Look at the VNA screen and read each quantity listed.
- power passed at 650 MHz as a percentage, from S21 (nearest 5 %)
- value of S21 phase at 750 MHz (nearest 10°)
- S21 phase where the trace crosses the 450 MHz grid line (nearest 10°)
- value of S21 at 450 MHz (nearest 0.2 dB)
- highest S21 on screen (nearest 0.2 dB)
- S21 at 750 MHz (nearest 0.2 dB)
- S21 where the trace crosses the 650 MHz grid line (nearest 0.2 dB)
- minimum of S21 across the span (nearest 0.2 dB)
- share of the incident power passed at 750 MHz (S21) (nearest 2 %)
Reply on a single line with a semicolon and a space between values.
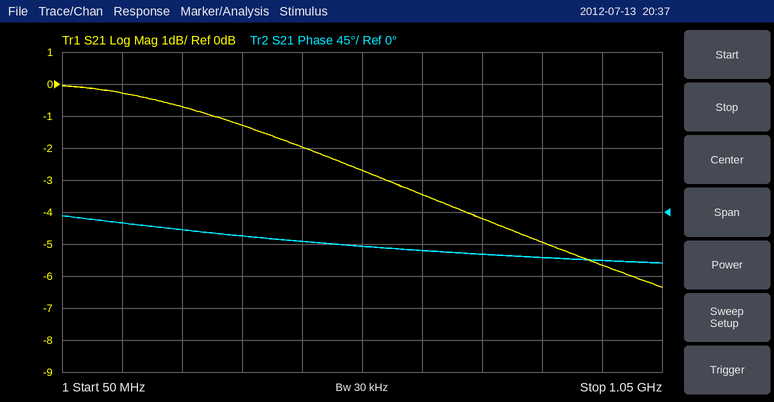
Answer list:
45 %; -60°; -40°; -2.0 dB; 0.0 dB; -4.2 dB; -3.4 dB; -6.4 dB; 38 %
